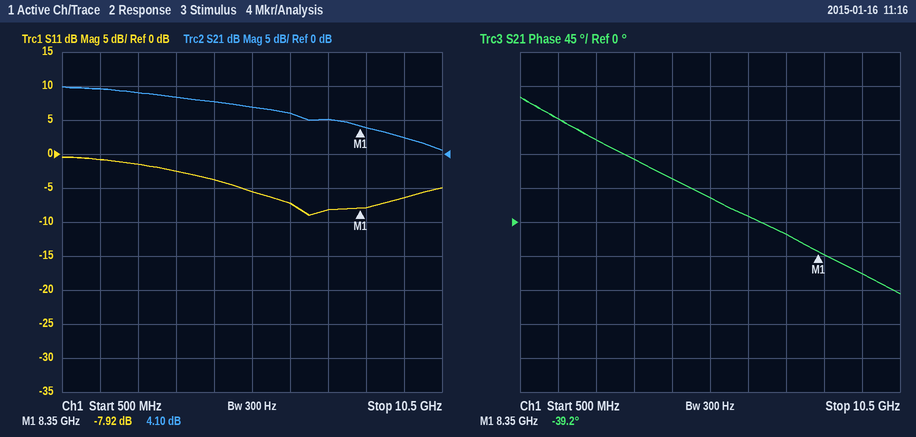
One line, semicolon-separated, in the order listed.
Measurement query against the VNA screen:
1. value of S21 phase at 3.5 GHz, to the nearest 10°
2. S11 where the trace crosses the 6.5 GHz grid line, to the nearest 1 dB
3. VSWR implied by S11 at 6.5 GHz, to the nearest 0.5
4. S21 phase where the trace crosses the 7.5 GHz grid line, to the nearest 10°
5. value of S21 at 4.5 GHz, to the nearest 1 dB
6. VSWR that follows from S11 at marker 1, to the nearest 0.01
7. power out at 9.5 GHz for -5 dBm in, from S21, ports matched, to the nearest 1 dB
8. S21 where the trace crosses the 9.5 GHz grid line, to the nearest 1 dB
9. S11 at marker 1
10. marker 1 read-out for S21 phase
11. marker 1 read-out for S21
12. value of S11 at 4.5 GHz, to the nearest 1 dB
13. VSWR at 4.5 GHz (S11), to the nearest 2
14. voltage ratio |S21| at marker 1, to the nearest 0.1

80°; -7 dB; 2.5; -20°; 8 dB; 2.34; -3 dBm; 2 dB; -7.92 dB; -39.2°; 4.10 dB; -4 dB; 4; 1.6
